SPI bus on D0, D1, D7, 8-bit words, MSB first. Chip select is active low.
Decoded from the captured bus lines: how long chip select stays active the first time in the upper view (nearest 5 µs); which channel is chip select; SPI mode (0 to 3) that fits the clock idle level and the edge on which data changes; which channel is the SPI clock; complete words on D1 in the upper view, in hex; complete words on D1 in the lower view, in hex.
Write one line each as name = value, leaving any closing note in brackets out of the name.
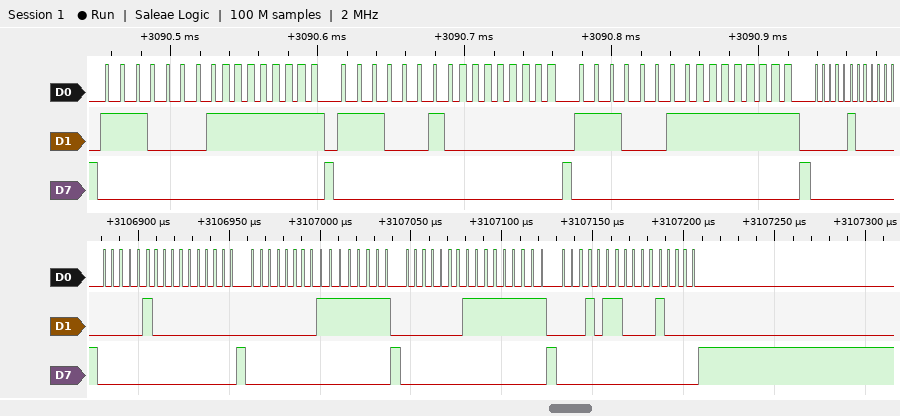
how long chip select stays active the first time in the upper view = 155 µs
which channel is chip select = D7
SPI mode (0 to 3) that fits the clock idle level and the edge on which data changes = 1
which channel is the SPI clock = D0
complete words on D1 in the upper view, in hex = E1, FF, E2, 00, E3, FF, 04
complete words on D1 in the lower view, in hex = 04, 00, 00, FF, 01, FF, 16, 10
